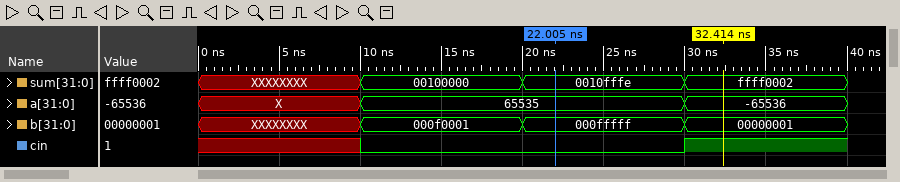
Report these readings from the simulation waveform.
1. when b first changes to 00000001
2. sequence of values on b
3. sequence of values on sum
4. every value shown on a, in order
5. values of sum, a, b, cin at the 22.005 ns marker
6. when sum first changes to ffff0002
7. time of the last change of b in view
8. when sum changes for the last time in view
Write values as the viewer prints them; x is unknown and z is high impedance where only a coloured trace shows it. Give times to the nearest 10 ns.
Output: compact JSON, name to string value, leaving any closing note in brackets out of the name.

{"when b first changes to 00000001": "30 ns", "sequence of values on b": "XXXXXXXX, 000f0001, 000fffff, 00000001", "sequence of values on sum": "XXXXXXXX, 00100000, 0010fffe, ffff0002", "every value shown on a, in order": "X, 65535, -65536", "values of sum, a, b, cin at the 22.005 ns marker": "sum=0010fffe, a=65535, b=000fffff, cin=0", "when sum first changes to ffff0002": "30 ns", "time of the last change of b in view": "30 ns", "when sum changes for the last time in view": "30 ns"}
